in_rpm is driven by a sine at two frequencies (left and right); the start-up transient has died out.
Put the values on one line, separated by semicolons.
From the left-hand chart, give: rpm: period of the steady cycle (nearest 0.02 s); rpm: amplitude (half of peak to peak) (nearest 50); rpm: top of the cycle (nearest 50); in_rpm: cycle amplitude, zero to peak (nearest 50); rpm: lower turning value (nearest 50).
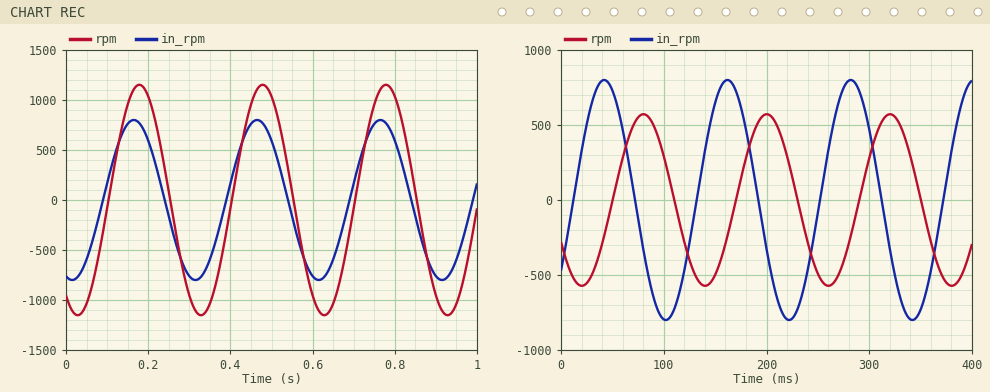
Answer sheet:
0.30 s; 1150; 1150; 800; -1150
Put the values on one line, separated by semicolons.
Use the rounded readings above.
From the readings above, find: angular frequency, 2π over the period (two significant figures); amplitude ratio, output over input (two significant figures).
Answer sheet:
21 rad/s; 1.4
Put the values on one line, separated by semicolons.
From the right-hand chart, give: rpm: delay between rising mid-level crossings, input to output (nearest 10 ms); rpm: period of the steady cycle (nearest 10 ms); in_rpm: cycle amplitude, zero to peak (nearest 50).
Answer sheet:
40 ms; 120 ms; 800
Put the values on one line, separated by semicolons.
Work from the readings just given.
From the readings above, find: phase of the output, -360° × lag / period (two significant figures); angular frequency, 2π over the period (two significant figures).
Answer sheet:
-120°; 0.052 rad/ms
